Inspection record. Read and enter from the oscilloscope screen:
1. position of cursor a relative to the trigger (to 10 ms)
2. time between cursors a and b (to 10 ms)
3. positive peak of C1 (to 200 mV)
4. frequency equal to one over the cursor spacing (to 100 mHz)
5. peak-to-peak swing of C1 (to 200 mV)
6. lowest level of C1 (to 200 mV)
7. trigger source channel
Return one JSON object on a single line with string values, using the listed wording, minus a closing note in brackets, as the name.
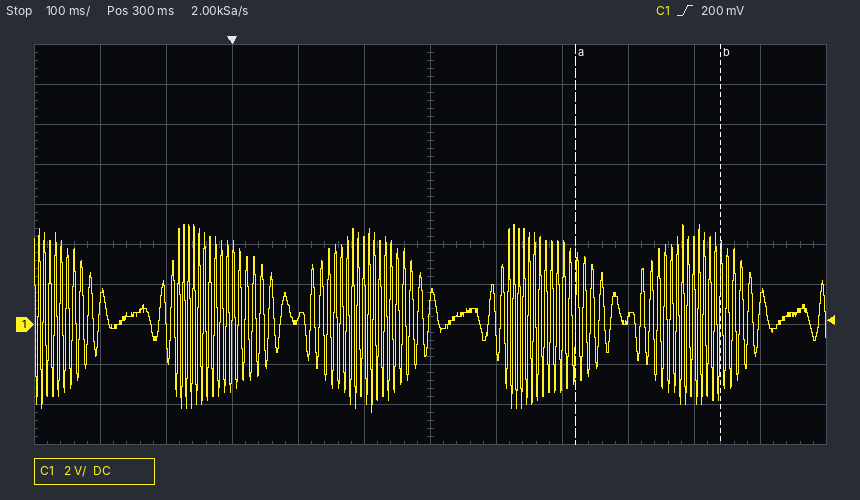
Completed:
{"position of cursor a relative to the trigger": "+520 ms", "time between cursors a and b": "220 ms", "positive peak of C1": "5.0 V", "frequency equal to one over the cursor spacing": "4.5 Hz", "peak-to-peak swing of C1": "9.4 V", "lowest level of C1": "-4.4 V", "trigger source channel": "C1"}
